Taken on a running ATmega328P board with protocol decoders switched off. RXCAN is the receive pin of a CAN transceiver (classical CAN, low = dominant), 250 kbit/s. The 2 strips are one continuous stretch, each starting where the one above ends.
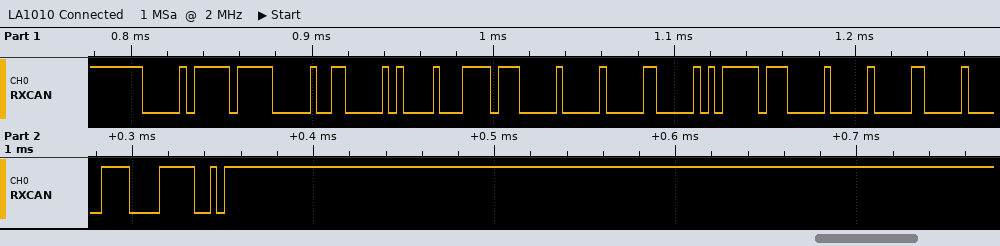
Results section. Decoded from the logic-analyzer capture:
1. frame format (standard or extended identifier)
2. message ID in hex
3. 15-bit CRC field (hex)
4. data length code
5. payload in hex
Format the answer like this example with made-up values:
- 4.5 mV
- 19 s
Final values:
- extended
- 0x00FF0302
- 0x1C3E
- 8
- F7 00 01 02 FF 00 01 00
